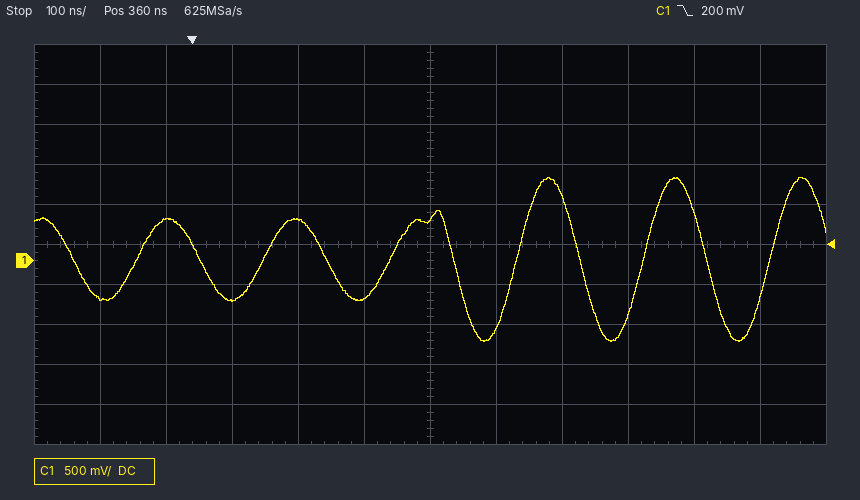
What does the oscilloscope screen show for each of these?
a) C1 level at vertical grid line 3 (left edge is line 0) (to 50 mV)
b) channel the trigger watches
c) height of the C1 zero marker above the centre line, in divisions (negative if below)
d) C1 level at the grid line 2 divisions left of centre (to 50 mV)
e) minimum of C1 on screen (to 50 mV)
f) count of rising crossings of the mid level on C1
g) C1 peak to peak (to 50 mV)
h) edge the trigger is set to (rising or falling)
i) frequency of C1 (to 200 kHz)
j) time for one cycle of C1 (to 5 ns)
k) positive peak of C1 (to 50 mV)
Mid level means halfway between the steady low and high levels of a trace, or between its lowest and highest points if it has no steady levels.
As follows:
-500 mV
C1
-0.4 div
500 mV
-1.00 V
6
2.05 V
falling
5.2 MHz
190 ns
1.05 V
